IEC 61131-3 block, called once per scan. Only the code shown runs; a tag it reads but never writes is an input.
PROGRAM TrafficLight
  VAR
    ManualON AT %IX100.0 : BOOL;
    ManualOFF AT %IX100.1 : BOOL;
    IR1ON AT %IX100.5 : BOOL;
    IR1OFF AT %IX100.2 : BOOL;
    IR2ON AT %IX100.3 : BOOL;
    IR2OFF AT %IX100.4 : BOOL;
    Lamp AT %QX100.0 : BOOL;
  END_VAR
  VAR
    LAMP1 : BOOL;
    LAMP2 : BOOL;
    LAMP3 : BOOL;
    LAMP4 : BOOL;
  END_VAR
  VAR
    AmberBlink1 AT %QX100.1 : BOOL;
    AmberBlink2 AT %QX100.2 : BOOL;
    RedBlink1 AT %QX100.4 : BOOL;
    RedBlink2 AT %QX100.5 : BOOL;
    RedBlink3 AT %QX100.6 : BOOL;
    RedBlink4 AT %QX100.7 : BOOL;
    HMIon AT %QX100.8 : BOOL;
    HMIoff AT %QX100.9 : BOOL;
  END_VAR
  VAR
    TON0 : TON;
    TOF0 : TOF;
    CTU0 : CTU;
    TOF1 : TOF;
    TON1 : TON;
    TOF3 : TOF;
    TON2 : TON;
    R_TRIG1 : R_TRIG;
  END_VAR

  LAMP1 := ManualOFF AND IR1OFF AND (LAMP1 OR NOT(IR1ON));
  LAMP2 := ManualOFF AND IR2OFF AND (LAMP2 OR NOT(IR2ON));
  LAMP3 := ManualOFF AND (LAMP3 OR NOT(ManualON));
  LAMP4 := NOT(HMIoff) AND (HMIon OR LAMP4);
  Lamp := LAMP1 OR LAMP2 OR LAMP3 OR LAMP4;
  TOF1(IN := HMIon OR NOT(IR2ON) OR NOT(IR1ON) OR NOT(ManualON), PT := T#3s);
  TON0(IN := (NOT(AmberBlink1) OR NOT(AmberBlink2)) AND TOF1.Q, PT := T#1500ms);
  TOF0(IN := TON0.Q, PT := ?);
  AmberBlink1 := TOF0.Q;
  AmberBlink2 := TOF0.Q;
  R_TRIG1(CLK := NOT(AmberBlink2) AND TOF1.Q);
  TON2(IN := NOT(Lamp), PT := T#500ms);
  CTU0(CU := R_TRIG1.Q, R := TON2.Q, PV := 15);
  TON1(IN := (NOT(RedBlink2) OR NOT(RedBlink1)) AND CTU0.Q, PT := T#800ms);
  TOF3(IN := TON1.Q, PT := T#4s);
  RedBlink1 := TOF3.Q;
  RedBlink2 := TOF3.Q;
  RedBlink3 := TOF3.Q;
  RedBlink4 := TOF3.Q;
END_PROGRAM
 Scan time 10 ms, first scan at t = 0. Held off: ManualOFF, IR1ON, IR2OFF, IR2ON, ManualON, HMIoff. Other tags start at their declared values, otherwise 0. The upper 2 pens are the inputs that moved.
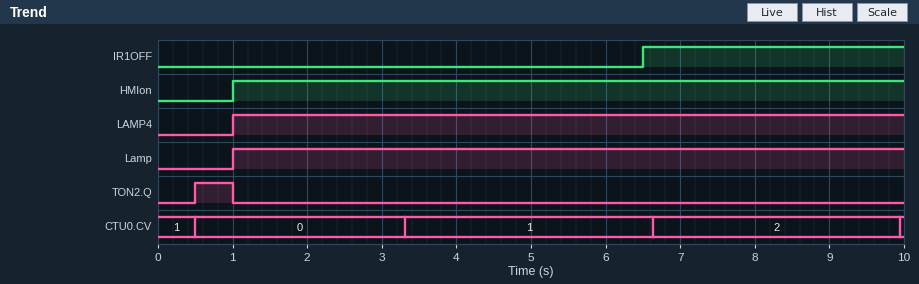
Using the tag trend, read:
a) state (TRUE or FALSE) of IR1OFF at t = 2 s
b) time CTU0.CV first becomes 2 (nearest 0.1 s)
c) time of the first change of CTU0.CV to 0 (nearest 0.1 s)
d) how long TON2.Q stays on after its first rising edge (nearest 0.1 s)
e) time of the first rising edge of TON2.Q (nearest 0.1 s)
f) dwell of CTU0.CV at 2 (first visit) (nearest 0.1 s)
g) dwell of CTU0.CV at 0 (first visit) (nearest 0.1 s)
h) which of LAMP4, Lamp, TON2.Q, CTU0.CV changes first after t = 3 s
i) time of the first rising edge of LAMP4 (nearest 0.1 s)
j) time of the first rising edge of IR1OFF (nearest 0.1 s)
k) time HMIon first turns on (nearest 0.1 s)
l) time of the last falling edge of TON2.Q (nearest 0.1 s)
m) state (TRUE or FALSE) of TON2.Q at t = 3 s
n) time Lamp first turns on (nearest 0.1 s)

FALSE
6.6 s
0.5 s
0.5 s
0.5 s
3.3 s
2.8 s
CTU0.CV
1.0 s
6.5 s
1.0 s
1.0 s
FALSE
1.0 s
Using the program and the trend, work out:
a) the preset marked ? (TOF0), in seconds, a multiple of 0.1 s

1.8 s
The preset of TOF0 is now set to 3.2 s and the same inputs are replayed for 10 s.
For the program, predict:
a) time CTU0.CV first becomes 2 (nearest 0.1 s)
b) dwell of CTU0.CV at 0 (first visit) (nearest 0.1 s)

9.4 s
4.2 s
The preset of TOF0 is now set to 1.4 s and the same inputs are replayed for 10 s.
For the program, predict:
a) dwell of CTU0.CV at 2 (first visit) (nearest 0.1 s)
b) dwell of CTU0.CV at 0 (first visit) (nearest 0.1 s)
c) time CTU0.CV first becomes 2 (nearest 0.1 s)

2.9 s
2.4 s
5.8 s
